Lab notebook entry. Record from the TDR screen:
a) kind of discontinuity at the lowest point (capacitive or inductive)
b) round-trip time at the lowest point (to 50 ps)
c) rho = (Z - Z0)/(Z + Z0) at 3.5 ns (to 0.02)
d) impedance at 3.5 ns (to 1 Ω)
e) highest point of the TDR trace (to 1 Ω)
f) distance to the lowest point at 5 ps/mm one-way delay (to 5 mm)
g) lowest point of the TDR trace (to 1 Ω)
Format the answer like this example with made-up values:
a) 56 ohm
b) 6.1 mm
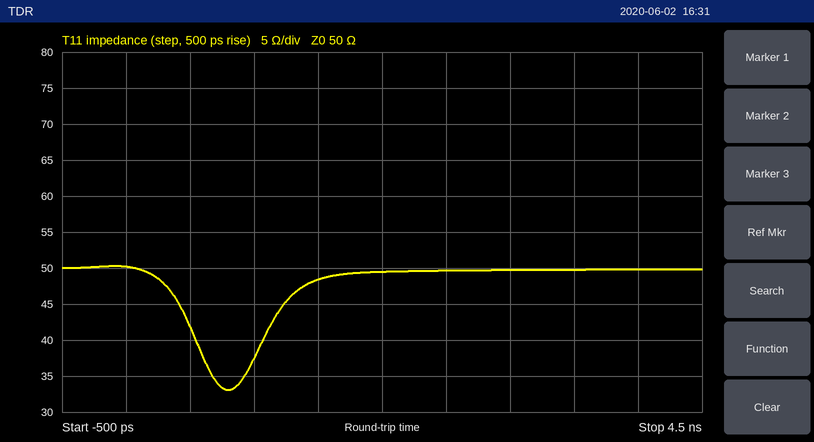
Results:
a) capacitive
b) 800 ps
c) 0.00
d) 50 Ω
e) 50 Ω
f) 80 mm
g) 33 Ω
